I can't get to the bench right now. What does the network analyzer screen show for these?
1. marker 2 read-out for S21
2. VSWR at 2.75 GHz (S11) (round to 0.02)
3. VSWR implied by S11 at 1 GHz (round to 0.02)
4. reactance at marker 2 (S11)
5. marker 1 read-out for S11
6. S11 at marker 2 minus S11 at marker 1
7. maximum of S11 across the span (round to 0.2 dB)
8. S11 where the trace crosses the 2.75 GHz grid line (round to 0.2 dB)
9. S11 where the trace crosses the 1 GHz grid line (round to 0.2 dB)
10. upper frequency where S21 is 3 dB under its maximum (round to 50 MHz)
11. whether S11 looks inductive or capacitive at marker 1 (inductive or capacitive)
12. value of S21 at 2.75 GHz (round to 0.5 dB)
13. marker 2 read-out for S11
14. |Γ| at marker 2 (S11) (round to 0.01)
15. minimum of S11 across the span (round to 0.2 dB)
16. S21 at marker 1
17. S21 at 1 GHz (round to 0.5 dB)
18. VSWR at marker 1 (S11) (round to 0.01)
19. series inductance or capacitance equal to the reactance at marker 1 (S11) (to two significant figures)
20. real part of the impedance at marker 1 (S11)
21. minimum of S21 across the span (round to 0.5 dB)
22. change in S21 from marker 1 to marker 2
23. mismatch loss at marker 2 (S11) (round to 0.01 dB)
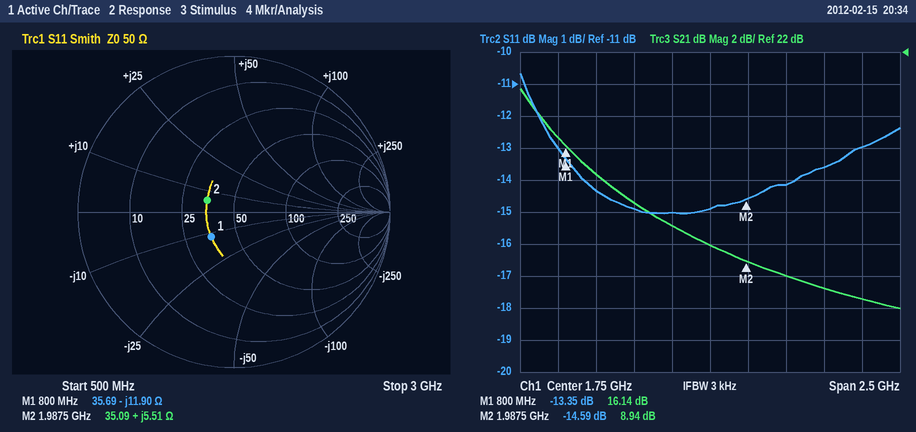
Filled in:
8.94 dB
1.58
1.48
+5.51 Ω
-13.35 dB
-1.24 dB
-10.6 dB
-13.0 dB
-14.4 dB
750 MHz
capacitive
6.5 dB
-14.59 dB
0.19
-15.0 dB
16.14 dB
14.5 dB
1.55
17 pF
35.69 Ω
6.0 dB
-7.20 dB
0.15 dB
